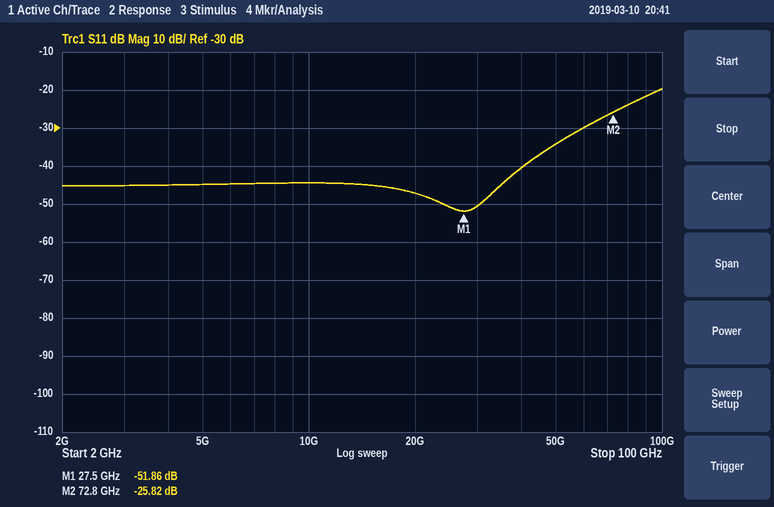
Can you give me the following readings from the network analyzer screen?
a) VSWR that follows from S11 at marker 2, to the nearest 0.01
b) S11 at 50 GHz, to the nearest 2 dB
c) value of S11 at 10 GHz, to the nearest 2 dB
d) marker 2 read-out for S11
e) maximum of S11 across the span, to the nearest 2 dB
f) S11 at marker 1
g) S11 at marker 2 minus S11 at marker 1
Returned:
1.11
-34 dB
-44 dB
-25.82 dB
-20 dB
-51.86 dB
26.04 dB
